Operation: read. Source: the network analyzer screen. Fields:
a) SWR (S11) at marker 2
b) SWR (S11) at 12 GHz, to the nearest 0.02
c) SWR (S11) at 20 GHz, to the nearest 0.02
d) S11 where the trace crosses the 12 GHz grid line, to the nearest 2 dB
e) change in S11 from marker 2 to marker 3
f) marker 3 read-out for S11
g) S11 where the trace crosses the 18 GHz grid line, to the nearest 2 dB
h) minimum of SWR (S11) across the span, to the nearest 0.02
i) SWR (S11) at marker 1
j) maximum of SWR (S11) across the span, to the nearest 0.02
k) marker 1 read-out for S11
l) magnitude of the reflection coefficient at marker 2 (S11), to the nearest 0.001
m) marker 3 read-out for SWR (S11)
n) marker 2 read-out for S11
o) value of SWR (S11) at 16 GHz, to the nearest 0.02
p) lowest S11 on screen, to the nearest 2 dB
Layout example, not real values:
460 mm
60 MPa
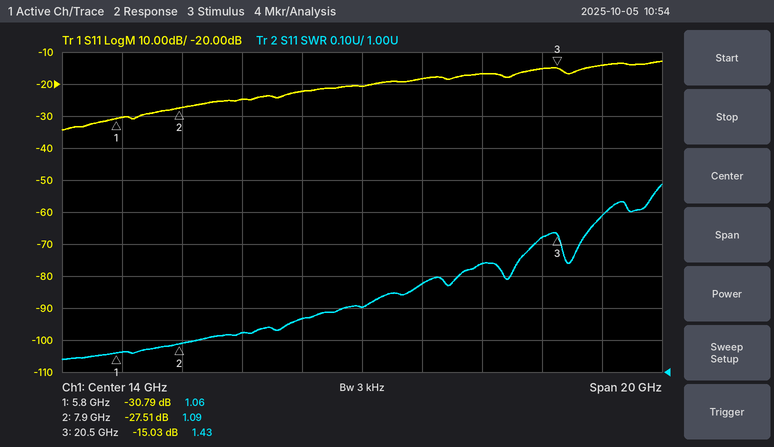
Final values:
1.09
1.16
1.42
-22 dB
12.48 dB
-15.03 dB
-16 dB
1.04
1.06
1.58
-30.79 dB
0.042
1.43
-27.51 dB
1.28
-34 dB
